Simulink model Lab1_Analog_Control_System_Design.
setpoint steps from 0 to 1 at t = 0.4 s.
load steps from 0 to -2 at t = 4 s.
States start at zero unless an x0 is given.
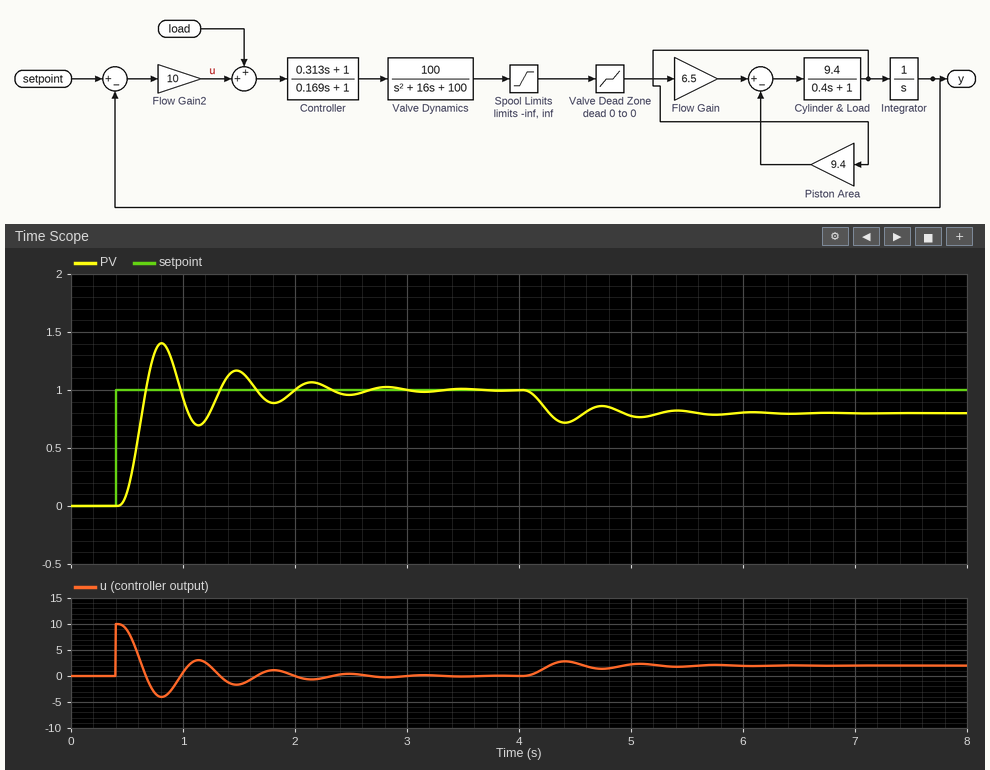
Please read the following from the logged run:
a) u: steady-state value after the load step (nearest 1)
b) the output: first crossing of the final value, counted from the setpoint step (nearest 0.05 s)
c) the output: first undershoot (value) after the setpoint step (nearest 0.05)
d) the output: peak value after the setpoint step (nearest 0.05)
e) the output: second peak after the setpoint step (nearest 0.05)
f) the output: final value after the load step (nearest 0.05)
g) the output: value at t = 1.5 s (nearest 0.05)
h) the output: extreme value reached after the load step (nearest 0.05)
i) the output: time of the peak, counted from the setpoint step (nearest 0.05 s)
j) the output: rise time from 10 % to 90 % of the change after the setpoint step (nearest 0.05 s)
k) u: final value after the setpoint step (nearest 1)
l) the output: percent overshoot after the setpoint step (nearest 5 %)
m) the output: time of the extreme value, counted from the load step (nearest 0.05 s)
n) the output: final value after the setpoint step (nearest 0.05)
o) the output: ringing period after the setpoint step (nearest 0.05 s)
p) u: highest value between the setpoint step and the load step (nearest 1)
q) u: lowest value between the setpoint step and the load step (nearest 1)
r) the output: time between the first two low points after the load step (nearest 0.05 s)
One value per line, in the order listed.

2
0.25 s
0.70
1.40
1.15
0.80
1.15
0.70
0.40 s
0.15 s
0
40 %
0.40 s
1.00
0.65 s
10
-4
0.65 s
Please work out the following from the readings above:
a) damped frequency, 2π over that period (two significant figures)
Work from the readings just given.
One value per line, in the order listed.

9.7 rad/s
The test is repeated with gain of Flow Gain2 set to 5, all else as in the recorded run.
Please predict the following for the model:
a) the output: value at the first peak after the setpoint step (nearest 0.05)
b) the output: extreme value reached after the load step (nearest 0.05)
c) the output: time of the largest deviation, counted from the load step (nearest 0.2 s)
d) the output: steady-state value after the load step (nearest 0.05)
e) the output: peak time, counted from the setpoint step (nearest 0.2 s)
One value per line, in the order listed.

1.05
0.60
0.6 s
0.60
0.6 s
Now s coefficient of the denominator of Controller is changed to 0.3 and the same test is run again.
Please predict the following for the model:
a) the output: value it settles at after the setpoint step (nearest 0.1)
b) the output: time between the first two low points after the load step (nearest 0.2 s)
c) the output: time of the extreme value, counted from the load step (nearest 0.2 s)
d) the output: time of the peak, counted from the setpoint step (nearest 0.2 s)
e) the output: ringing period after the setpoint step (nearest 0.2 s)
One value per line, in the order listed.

1.0
0.8 s
0.6 s
0.6 s
0.8 s
